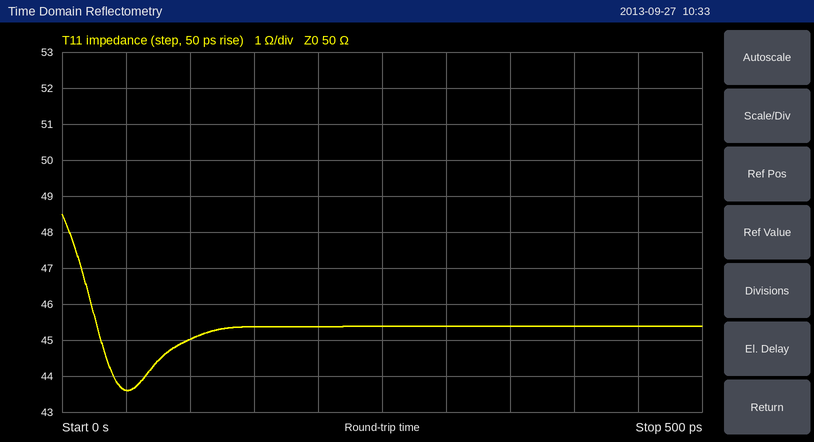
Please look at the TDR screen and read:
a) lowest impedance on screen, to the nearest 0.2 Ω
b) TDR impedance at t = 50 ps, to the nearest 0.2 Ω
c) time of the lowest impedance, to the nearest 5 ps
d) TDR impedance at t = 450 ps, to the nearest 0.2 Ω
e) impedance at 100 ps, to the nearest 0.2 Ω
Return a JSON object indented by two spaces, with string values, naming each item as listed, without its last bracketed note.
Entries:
{
  "lowest impedance on screen, to the nearest 0.2 Ω": "43.6 Ω",
  "TDR impedance at t = 50 ps, to the nearest 0.2 Ω": "43.6 Ω",
  "time of the lowest impedance, to the nearest 5 ps": "50 ps",
  "TDR impedance at t = 450 ps, to the nearest 0.2 Ω": "45.4 Ω",
  "impedance at 100 ps, to the nearest 0.2 Ω": "45.0 Ω"
}
